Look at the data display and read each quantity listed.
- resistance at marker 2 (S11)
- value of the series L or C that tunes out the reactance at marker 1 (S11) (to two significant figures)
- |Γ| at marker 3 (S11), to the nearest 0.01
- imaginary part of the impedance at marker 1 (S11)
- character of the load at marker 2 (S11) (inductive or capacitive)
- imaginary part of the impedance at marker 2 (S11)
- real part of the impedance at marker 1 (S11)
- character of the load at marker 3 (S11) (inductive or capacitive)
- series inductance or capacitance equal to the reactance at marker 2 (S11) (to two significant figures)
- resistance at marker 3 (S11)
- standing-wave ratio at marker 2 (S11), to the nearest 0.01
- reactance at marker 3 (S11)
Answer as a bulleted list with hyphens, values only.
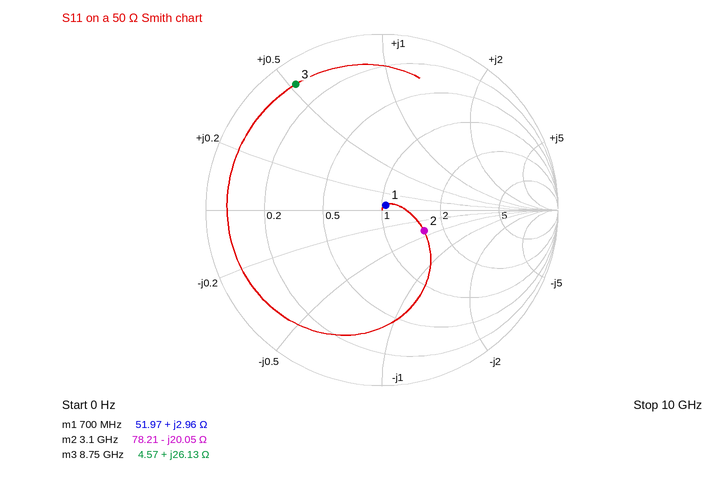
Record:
- 78.21 Ω
- 77 pF
- 0.87
- +2.96 Ω
- capacitive
- -20.05 Ω
- 51.97 Ω
- inductive
- 2.6 pF
- 4.57 Ω
- 1.73
- +26.13 Ω
